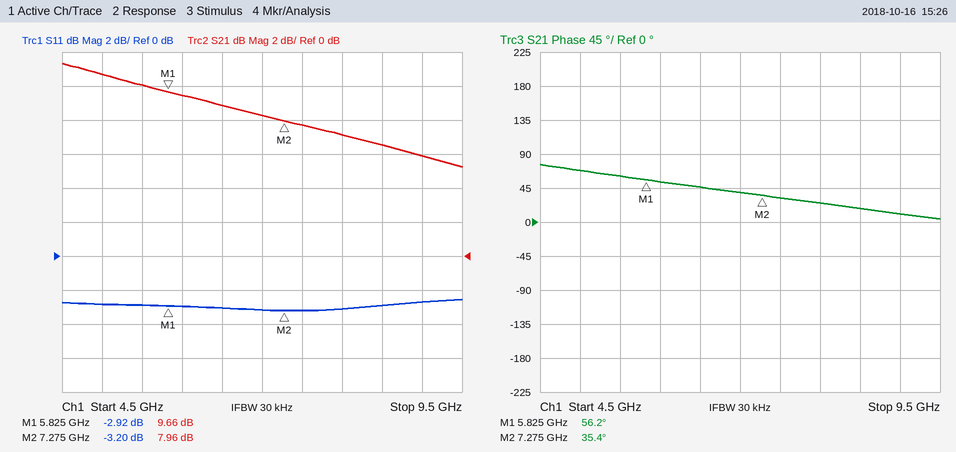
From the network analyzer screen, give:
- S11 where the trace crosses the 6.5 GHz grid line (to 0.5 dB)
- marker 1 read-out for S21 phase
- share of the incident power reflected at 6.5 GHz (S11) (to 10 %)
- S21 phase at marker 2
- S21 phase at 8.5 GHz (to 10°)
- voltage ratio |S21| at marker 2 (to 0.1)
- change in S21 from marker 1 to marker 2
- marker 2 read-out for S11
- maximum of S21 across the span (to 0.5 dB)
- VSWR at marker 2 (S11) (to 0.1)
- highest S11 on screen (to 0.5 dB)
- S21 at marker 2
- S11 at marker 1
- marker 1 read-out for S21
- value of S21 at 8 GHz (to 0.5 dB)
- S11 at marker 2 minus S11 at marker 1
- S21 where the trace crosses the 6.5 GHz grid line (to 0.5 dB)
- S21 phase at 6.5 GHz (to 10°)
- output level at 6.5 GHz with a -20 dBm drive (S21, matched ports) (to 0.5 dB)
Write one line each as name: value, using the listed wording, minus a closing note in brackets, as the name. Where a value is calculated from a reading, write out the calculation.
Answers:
S11 where the trace crosses the 6.5 GHz grid line: -3.0 dB
marker 1 read-out for S21 phase: 56.2°
share of the incident power reflected at 6.5 GHz (S11): 10^(-3/10) ≈ 50 %
S21 phase at marker 2: 35.4°
S21 phase at 8.5 GHz: 20°
voltage ratio |S21| at marker 2: 10^(7.96/20) ≈ 2.5
change in S21 from marker 1 to marker 2: 7.96 − (9.66) = -1.70 dB
marker 2 read-out for S11: -3.20 dB
maximum of S21 across the span: 11.5 dB
VSWR at marker 2 (S11): (1 + 0.6918)/(1 − 0.6918) ≈ 5.5
highest S11 on screen: -2.5 dB
S21 at marker 2: 7.96 dB
S11 at marker 1: -2.92 dB
marker 1 read-out for S21: 9.66 dB
value of S21 at 8 GHz: 7.0 dB
S11 at marker 2 minus S11 at marker 1: -3.2 − (-2.92) = -0.28 dB
S21 where the trace crosses the 6.5 GHz grid line: 9.0 dB
S21 phase at 6.5 GHz: 50°
output level at 6.5 GHz with a -20 dBm drive (S21, matched ports): -20 dBm + (9.0 dB) = -11.0 dBm
